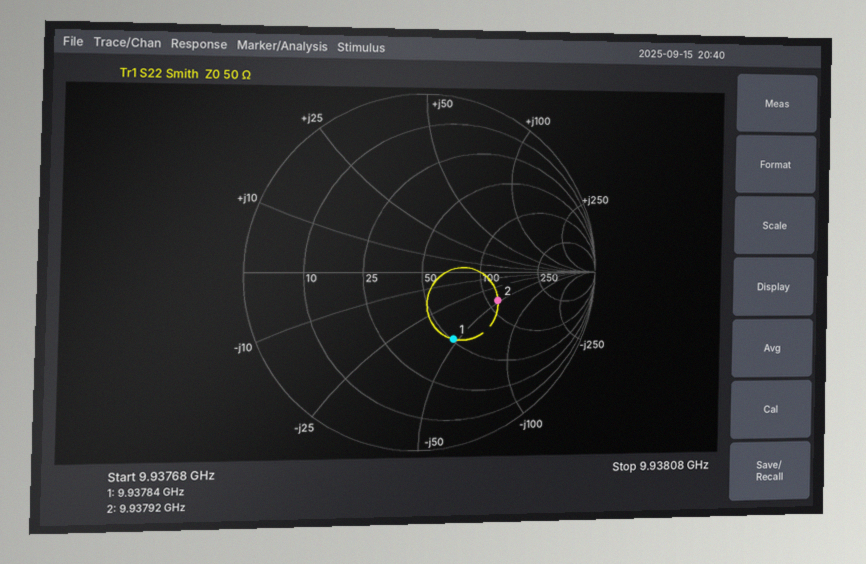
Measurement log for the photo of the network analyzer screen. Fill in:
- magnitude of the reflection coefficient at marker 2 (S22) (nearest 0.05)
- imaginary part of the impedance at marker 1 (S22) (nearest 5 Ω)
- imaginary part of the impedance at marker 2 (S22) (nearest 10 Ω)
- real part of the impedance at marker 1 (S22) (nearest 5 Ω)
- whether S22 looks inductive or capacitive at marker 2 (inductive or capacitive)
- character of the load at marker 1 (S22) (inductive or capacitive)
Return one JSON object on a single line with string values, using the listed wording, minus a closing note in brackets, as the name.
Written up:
{"magnitude of the reflection coefficient at marker 2 (S22)": "0.45", "imaginary part of the impedance at marker 1 (S22)": "-45 Ω", "imaginary part of the impedance at marker 2 (S22)": "-50 Ω", "real part of the impedance at marker 1 (S22)": "50 Ω", "whether S22 looks inductive or capacitive at marker 2": "capacitive", "character of the load at marker 1 (S22)": "capacitive"}
